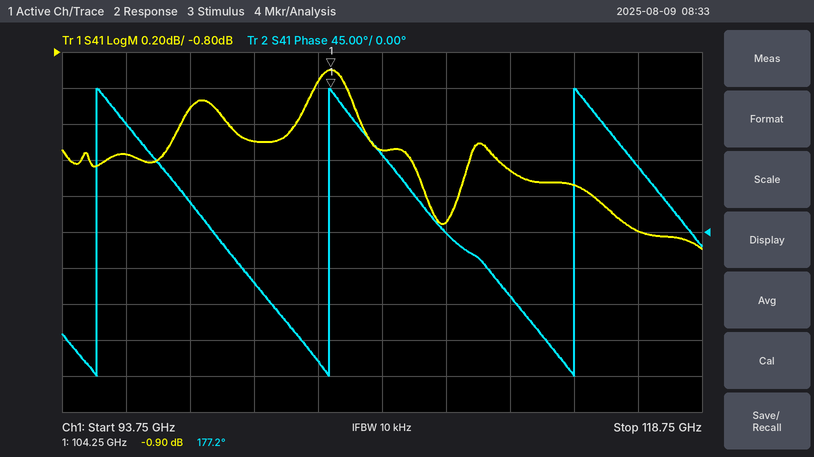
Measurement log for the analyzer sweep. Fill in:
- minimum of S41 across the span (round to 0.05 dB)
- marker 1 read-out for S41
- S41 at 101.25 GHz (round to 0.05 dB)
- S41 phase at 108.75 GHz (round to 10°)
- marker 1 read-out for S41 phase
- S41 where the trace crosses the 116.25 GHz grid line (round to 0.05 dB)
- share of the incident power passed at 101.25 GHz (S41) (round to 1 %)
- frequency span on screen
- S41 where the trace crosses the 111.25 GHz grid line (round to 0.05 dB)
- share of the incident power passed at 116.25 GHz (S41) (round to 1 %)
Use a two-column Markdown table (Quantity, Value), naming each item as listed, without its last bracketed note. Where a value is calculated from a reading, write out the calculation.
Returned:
| Quantity | Value |
|---|---|
| minimum of S41 across the span | -1.90 dB |
| marker 1 read-out for S41 | -0.90 dB |
| S41 at 101.25 GHz | -1.30 dB |
| S41 phase at 108.75 GHz | 0° |
| marker 1 read-out for S41 phase | 177.2° |
| S41 where the trace crosses the 116.25 GHz grid line | -1.80 dB |
| share of the incident power passed at 101.25 GHz (S41) | 10^(-1.3/10) ≈ 74 % |
| frequency span on screen | 25 GHz |
| S41 where the trace crosses the 111.25 GHz grid line | -1.45 dB |
| share of the incident power passed at 116.25 GHz (S41) | 10^(-1.8/10) ≈ 66 % |
